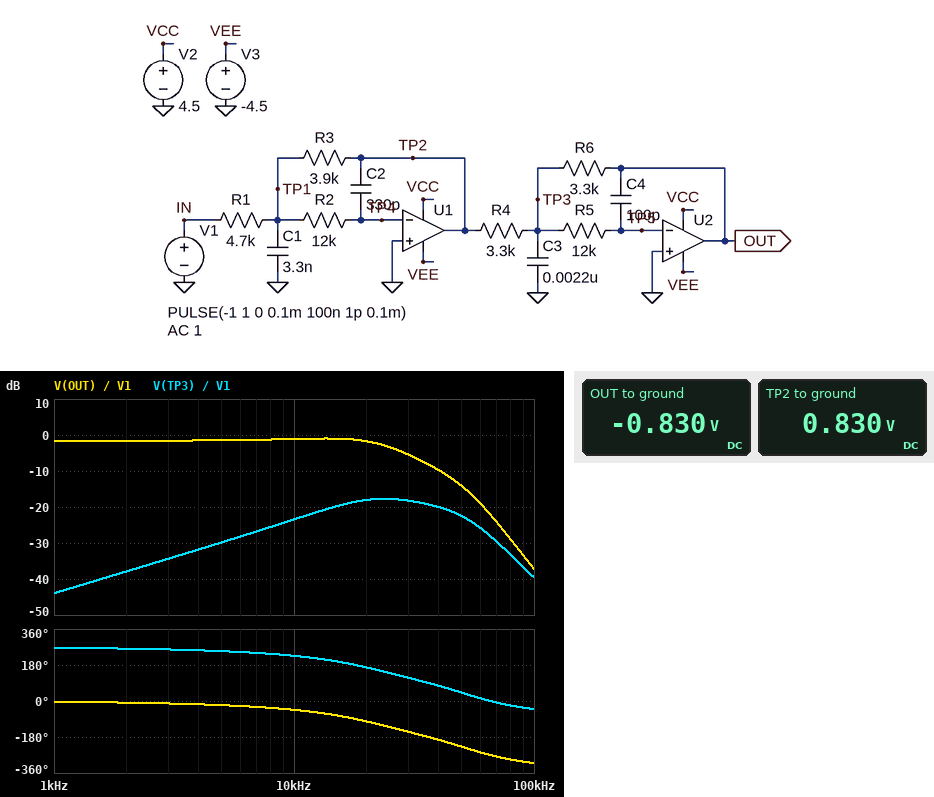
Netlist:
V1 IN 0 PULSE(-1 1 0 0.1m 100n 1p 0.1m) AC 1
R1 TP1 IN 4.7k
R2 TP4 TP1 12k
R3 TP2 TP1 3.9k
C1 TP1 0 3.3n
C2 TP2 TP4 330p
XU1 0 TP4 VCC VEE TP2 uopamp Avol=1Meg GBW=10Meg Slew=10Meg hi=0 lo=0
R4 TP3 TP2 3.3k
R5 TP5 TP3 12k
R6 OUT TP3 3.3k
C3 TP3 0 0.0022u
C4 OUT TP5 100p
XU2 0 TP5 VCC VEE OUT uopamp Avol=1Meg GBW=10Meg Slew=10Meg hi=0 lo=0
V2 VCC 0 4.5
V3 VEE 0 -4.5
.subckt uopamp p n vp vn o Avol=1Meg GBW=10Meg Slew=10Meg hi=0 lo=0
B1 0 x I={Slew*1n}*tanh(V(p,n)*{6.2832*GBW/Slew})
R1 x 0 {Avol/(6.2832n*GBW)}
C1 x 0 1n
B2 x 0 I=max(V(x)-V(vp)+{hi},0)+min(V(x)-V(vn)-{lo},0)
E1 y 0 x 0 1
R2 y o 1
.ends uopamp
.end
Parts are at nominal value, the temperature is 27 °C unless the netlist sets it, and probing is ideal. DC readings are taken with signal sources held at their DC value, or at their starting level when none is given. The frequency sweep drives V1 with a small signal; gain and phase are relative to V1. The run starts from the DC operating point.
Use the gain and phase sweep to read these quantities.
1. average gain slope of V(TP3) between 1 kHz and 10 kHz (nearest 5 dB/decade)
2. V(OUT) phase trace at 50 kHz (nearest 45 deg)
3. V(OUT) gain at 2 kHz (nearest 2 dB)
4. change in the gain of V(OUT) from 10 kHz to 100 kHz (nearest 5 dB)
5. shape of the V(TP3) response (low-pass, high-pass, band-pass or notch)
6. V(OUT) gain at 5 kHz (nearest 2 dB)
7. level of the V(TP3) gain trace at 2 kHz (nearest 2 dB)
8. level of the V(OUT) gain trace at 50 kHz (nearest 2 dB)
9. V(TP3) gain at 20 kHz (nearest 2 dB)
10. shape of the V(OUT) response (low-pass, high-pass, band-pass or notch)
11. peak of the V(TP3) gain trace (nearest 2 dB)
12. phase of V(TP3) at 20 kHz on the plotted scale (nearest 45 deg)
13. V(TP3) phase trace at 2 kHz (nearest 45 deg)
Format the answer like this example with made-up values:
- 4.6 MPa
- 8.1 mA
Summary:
- 20 dB/decade
- -225 deg
- -2 dB
- -35 dB
- band-pass
- -2 dB
- -38 dB
- -14 dB
- -18 dB
- low-pass
- -18 dB
- 180 deg
- 270 deg
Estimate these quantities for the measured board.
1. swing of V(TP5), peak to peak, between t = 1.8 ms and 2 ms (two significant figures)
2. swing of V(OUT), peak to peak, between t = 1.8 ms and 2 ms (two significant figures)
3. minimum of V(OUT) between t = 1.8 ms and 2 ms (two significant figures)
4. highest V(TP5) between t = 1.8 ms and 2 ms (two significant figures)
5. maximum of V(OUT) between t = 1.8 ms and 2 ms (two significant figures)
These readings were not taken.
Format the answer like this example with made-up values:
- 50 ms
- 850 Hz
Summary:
- 2.3 mV
- 1.4 V
- -750 mV
- 1.8 mV
- 680 mV
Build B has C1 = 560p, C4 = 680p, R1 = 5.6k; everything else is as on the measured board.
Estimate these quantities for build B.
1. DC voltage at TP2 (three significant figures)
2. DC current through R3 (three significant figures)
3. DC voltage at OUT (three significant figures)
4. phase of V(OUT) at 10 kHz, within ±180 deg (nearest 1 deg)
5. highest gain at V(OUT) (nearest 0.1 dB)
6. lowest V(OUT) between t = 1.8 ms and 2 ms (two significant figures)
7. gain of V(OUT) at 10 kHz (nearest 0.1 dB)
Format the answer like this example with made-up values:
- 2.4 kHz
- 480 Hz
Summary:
- 696 mV
- 179 µA
- -696 mV
- -84 deg
- -3.1 dB
- -270 mV
- -6.8 dB
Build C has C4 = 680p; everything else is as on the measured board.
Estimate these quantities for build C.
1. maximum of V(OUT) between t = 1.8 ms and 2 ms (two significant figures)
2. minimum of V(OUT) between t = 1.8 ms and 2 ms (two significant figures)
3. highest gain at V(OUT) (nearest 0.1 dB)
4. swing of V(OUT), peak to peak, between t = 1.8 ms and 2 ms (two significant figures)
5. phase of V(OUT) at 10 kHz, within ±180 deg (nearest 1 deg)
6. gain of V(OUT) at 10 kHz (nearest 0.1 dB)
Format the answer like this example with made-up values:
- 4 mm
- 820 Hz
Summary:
- 470 mV
- -400 mV
- -1.6 dB
- 870 mV
- -91 deg
- -4.2 dB
